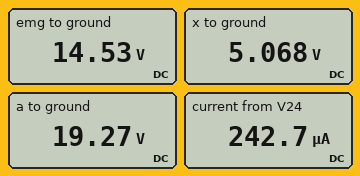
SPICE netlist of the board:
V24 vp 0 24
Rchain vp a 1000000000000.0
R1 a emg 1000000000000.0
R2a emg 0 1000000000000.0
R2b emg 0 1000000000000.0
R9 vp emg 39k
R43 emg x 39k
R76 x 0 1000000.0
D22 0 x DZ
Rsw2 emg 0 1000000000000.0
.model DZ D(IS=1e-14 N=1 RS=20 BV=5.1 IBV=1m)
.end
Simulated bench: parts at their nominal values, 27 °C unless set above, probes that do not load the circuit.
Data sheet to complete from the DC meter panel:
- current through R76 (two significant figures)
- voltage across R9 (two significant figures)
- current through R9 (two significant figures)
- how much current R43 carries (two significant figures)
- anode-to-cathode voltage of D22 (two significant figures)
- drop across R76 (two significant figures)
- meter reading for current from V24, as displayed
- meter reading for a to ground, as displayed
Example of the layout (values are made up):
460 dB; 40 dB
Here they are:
5.1 µA; 9.5 V; 240 µA; 240 µA; -5.1 V; 5.1 V; 242.7 µA; 19.27 V
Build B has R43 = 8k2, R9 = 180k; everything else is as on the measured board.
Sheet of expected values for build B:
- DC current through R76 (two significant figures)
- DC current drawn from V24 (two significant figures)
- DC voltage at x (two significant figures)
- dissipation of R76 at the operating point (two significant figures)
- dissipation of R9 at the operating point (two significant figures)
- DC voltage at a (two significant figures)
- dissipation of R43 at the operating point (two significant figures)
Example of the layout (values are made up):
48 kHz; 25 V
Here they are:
5.0 µA; 100 µA; 5.0 V; 25 µW; 1.8 mW; 15 V; 83 µW
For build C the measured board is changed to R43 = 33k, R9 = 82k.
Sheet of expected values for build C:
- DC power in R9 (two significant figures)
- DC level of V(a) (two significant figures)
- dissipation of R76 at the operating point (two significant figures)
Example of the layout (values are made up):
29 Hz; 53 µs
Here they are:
2.2 mW; 17 V; 26 µW
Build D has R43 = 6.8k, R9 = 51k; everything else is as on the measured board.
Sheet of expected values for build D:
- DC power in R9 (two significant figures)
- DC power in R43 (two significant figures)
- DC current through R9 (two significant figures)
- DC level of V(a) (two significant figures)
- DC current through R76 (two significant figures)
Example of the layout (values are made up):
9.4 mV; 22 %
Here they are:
5.5 mW; 730 µW; 330 µA; 16 V; 5.1 µA
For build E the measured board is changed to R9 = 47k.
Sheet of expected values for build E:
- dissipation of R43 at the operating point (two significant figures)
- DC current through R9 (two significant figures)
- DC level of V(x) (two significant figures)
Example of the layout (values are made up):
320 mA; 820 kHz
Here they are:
1.9 mW; 220 µA; 5.1 V
